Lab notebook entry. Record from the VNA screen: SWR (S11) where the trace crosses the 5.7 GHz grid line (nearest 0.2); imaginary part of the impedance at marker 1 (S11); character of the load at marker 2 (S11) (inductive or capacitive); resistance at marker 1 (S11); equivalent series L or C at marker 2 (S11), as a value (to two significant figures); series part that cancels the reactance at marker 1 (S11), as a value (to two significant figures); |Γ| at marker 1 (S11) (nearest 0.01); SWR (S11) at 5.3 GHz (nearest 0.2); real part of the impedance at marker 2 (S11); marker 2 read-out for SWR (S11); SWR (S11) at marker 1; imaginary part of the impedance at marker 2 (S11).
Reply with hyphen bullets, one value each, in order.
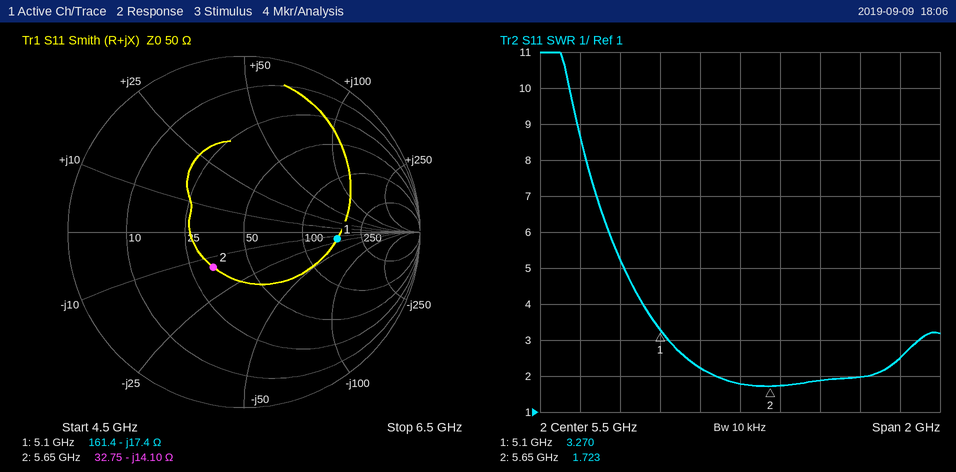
- 1.8
- -17.4 Ω
- capacitive
- 161.4 Ω
- 2.0 pF
- 540 pH
- 0.53
- 2.2
- 32.75 Ω
- 1.723
- 3.270
- -14.10 Ω
